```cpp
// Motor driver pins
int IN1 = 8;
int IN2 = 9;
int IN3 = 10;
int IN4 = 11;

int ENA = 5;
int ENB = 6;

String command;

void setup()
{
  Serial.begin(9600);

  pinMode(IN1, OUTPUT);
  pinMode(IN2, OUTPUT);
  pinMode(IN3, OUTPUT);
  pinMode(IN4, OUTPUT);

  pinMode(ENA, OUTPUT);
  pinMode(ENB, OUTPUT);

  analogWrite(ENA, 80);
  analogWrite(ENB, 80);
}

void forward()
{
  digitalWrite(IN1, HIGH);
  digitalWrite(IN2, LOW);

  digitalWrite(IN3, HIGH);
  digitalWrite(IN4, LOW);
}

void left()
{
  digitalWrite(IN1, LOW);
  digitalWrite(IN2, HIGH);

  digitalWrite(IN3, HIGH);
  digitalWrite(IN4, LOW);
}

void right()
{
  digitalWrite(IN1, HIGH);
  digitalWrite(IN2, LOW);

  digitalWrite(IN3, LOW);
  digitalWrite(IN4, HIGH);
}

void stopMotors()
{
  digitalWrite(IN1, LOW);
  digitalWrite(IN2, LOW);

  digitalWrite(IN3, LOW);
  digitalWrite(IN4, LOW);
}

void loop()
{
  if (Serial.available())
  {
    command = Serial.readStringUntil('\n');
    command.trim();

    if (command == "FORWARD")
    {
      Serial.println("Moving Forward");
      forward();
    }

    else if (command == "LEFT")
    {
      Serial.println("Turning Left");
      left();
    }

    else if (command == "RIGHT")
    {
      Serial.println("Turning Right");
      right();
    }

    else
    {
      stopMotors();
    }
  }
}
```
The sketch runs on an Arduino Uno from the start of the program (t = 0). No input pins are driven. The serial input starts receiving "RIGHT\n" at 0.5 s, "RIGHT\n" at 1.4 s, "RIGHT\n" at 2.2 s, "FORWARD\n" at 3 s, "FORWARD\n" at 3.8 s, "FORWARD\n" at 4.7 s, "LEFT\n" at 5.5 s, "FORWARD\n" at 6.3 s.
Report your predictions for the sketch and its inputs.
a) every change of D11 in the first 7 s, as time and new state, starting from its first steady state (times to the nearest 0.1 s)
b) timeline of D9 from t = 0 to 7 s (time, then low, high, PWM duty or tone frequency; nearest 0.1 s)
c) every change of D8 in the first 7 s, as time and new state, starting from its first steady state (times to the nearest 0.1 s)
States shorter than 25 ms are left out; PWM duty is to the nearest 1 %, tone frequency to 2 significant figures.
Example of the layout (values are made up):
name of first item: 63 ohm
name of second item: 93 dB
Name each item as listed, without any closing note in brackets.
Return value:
every change of D11 in the first 7 s, as time and new state, starting from its first steady state: 0 s low; 0.5 s high; 3 s low
timeline of D9 from t = 0 to 7 s: 0 s low; 5.5 s high; 6.3 s low
every change of D8 in the first 7 s, as time and new state, starting from its first steady state: 0 s low; 0.5 s high; 5.5 s low; 6.3 s high
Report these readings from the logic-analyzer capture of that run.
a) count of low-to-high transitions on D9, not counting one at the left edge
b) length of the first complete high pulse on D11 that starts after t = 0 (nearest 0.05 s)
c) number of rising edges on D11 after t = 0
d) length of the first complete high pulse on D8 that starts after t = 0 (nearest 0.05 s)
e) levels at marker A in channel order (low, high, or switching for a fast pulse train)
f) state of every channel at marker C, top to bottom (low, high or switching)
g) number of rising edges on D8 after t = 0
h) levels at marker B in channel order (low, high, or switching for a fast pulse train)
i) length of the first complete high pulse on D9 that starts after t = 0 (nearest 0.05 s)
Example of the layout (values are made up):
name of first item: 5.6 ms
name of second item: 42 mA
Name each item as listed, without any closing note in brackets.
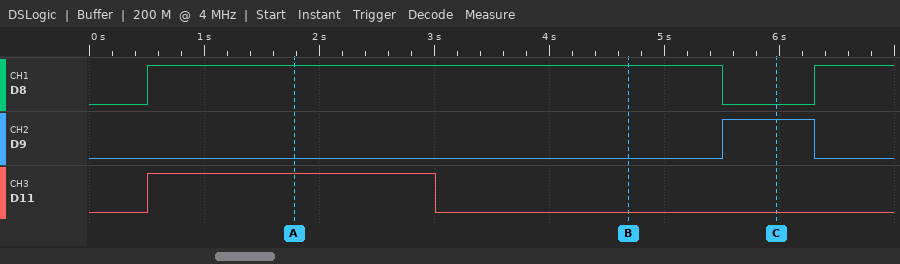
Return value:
count of low-to-high transitions on D9, not counting one at the left edge: 1
length of the first complete high pulse on D11 that starts after t = 0: 2.50 s
number of rising edges on D11 after t = 0: 1
length of the first complete high pulse on D8 that starts after t = 0: 5.00 s
levels at marker A in channel order: D8 high, D9 low, D11 high
state of every channel at marker C, top to bottom: D8 low, D9 high, D11 low
number of rising edges on D8 after t = 0: 2
levels at marker B in channel order: D8 high, D9 low, D11 low
length of the first complete high pulse on D9 that starts after t = 0: 0.80 s
